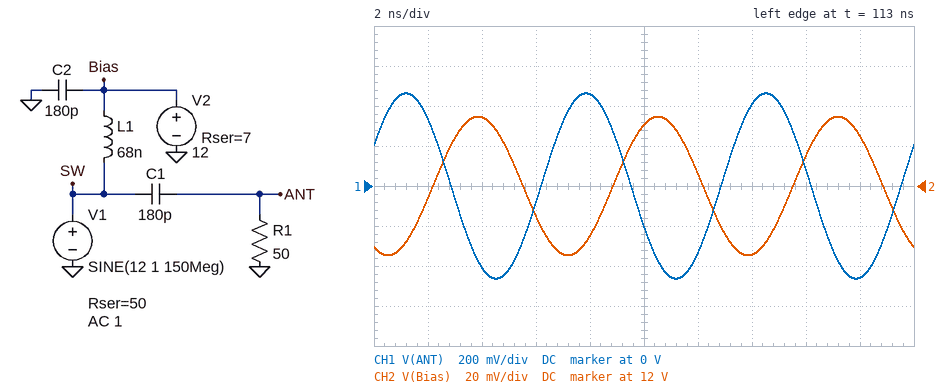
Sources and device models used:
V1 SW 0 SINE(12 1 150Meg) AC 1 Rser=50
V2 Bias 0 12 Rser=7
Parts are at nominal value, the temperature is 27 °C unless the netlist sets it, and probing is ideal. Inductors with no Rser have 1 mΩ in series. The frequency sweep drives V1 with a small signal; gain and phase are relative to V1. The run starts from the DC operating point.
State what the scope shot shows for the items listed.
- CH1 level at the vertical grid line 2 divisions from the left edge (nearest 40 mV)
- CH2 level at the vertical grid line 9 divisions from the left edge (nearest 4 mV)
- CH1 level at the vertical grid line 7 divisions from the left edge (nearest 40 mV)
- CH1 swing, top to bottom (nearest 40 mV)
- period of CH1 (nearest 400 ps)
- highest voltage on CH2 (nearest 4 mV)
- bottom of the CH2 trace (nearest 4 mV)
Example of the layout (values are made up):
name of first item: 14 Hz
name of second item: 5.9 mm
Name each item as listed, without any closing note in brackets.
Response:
CH1 level at the vertical grid line 2 divisions from the left edge: -400 mV
CH2 level at the vertical grid line 9 divisions from the left edge: 12.024 V
CH1 level at the vertical grid line 7 divisions from the left edge: 400 mV
CH1 swing, top to bottom: 920 mV
period of CH1: 6.8 ns
highest voltage on CH2: 12.036 V
bottom of the CH2 trace: 11.964 V
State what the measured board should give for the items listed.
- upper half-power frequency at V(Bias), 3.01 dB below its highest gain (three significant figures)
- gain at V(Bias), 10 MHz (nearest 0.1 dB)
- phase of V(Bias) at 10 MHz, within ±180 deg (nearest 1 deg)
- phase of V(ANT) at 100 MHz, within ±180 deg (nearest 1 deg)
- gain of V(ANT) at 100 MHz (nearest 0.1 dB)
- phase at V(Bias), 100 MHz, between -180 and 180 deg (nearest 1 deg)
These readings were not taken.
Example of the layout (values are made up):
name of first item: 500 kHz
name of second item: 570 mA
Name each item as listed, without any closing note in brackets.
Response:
upper half-power frequency at V(Bias), 3.01 dB below its highest gain: 62.3 MHz
gain at V(Bias), 10 MHz: -18.3 dB
phase of V(Bias) at 10 MHz, within ±180 deg: -12 deg
phase of V(ANT) at 100 MHz, within ±180 deg: 37 deg
gain of V(ANT) at 100 MHz: -7.6 dB
phase at V(Bias), 100 MHz, between -180 and 180 deg: -95 deg
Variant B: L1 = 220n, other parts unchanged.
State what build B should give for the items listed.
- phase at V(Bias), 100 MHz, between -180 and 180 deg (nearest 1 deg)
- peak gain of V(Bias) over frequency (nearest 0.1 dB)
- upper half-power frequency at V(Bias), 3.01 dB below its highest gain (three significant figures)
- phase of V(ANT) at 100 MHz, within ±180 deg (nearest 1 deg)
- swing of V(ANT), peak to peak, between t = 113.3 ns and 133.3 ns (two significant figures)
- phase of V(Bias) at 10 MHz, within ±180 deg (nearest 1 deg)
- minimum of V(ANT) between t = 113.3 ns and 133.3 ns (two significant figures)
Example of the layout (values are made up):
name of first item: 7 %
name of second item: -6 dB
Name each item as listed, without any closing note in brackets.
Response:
phase at V(Bias), 100 MHz, between -180 and 180 deg: -121 deg
peak gain of V(Bias) over frequency: -18.1 dB
upper half-power frequency at V(Bias), 3.01 dB below its highest gain: 26.8 MHz
phase of V(ANT) at 100 MHz, within ±180 deg: 16 deg
swing of V(ANT), peak to peak, between t = 113.3 ns and 133.3 ns: 1.0 V
phase of V(Bias) at 10 MHz, within ±180 deg: -25 deg
minimum of V(ANT) between t = 113.3 ns and 133.3 ns: -500 mV
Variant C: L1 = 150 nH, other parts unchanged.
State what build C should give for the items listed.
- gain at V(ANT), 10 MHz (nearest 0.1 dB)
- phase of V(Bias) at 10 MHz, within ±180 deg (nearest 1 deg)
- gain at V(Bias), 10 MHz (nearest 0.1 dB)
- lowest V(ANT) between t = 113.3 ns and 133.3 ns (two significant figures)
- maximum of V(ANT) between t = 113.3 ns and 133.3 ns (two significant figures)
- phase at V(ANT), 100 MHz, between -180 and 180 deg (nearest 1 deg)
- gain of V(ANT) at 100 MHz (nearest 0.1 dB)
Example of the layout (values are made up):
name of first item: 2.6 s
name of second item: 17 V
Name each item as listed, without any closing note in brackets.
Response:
gain at V(ANT), 10 MHz: -20.2 dB
phase of V(Bias) at 10 MHz, within ±180 deg: -19 deg
gain at V(Bias), 10 MHz: -18.2 dB
lowest V(ANT) between t = 113.3 ns and 133.3 ns: -490 mV
maximum of V(ANT) between t = 113.3 ns and 133.3 ns: 490 mV
phase at V(ANT), 100 MHz, between -180 and 180 deg: 21 deg
gain of V(ANT) at 100 MHz: -6.3 dB
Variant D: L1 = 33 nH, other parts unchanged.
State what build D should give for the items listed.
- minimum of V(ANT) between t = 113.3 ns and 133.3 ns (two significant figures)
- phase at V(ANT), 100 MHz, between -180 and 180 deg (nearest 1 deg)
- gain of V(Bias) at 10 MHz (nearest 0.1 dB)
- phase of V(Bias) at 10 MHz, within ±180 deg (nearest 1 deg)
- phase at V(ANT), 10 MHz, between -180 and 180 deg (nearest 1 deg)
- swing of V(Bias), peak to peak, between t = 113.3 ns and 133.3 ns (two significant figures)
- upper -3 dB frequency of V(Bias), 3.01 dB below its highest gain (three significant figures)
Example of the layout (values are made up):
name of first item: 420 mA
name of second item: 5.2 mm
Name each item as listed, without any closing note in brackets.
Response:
minimum of V(ANT) between t = 113.3 ns and 133.3 ns: -360 mV
phase at V(ANT), 100 MHz, between -180 and 180 deg: 54 deg
gain of V(Bias) at 10 MHz: -18.4 dB
phase of V(Bias) at 10 MHz, within ±180 deg: -9 deg
phase at V(ANT), 10 MHz, between -180 and 180 deg: 68 deg
swing of V(Bias), peak to peak, between t = 113.3 ns and 133.3 ns: 120 mV
upper -3 dB frequency of V(Bias), 3.01 dB below its highest gain: 93.9 MHz
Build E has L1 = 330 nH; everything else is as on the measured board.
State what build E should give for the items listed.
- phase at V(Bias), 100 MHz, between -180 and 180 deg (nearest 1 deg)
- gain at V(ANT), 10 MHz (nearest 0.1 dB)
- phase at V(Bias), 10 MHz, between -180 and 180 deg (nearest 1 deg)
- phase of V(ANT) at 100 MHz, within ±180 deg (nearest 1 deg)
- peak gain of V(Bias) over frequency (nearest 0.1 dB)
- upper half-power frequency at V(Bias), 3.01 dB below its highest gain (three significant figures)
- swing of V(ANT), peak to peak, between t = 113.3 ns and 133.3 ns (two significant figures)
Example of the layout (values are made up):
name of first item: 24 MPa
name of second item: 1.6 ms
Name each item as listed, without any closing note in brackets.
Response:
phase at V(Bias), 100 MHz, between -180 and 180 deg: -125 deg
gain at V(ANT), 10 MHz: -14.7 dB
phase at V(Bias), 10 MHz, between -180 and 180 deg: -34 deg
phase of V(ANT) at 100 MHz, within ±180 deg: 12 deg
peak gain of V(Bias) over frequency: -18.1 dB
upper half-power frequency at V(Bias), 3.01 dB below its highest gain: 20.2 MHz
swing of V(ANT), peak to peak, between t = 113.3 ns and 133.3 ns: 1.0 V
